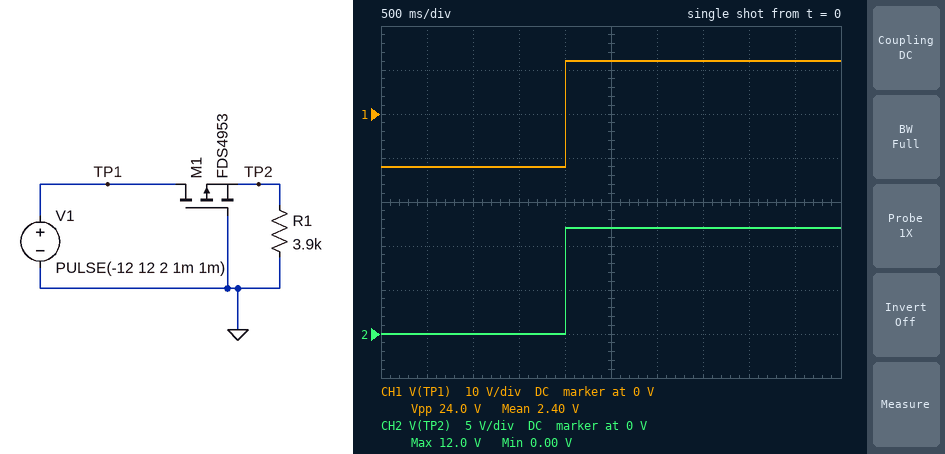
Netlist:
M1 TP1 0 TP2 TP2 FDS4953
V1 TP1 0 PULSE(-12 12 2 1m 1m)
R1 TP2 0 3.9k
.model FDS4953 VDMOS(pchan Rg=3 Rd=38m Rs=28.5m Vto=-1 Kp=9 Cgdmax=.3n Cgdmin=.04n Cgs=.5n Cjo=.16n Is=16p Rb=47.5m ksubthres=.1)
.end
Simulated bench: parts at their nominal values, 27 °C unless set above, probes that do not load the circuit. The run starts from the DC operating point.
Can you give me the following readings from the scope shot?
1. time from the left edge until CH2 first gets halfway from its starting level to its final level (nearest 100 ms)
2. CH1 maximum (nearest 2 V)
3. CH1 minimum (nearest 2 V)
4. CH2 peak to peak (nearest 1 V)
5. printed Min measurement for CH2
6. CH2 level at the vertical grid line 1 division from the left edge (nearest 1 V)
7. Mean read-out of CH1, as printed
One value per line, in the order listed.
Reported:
2.0 s
12 V
-12 V
12 V
0.00 V
0 V
2.40 V
